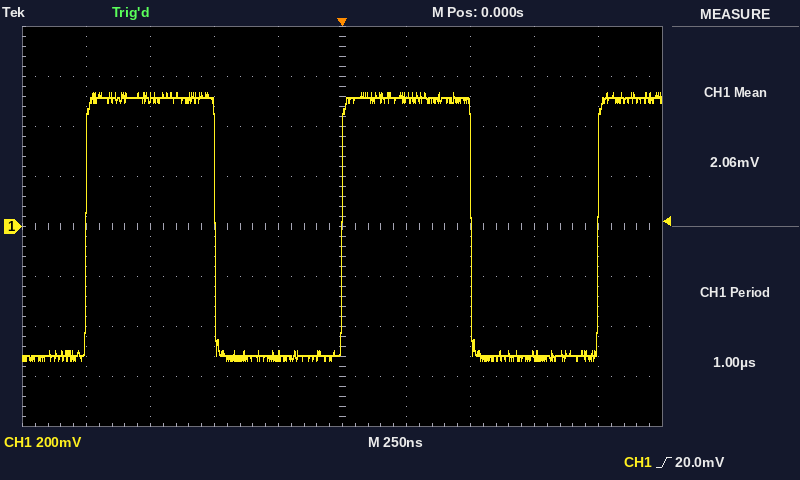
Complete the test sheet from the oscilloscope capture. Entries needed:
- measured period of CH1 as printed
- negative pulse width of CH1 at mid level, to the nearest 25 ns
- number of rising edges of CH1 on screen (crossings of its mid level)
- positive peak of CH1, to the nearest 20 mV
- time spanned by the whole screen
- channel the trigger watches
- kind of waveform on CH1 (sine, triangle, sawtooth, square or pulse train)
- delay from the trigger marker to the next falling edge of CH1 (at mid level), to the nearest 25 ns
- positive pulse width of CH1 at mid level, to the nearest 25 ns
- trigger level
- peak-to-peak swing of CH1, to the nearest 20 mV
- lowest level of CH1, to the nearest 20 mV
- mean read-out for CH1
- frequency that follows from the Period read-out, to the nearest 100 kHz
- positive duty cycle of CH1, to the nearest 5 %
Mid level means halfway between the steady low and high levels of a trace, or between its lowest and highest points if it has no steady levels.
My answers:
1.00 µs
500 ns
3
540 mV
2.5 µs
CH1
square
500 ns
500 ns
20.0 mV
1.08 V
-540 mV
2.06 mV
1.0 MHz
50 %
